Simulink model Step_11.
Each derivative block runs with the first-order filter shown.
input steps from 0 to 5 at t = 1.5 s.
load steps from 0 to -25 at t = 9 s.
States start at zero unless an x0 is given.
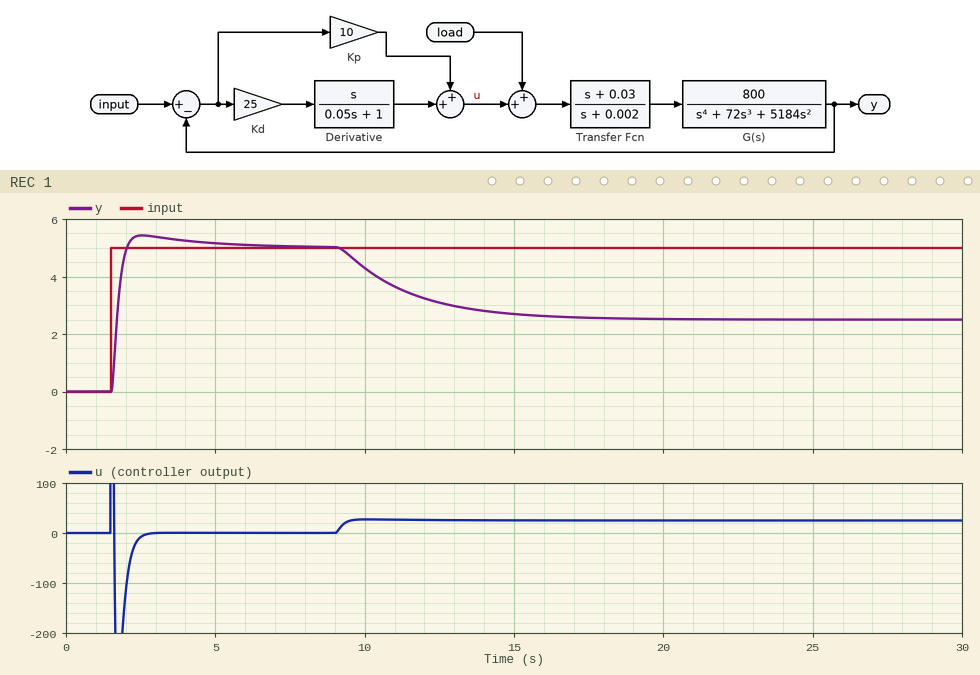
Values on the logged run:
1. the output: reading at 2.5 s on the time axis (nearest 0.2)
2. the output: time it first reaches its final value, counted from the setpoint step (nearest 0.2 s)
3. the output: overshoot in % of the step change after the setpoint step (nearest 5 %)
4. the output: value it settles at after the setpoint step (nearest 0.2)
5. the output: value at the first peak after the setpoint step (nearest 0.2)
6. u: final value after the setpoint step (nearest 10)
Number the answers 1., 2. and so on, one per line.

1. 5.4
2. 0.6 s
3. 10 %
4. 5.0
5. 5.4
6. 0
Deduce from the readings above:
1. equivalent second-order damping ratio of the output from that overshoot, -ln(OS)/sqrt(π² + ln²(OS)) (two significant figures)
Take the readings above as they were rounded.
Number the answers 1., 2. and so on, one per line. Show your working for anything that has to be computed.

1. ln(0.1) = -2.303; 2.303 / sqrt(9.870 + 5.302) = 0.59
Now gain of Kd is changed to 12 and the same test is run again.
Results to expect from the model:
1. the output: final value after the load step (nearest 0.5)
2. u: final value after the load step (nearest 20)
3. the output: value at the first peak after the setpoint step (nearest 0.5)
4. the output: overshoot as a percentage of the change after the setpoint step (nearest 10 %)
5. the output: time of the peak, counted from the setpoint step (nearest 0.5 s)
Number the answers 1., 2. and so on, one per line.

1. 2.5
2. 20
3. 6.0
4. 20 %
5. 1.5 s
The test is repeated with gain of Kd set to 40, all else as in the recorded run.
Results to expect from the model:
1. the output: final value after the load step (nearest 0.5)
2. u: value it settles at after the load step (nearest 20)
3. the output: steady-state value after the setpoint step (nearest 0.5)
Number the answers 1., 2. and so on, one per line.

1. 2.5
2. 20
3. 5.0
